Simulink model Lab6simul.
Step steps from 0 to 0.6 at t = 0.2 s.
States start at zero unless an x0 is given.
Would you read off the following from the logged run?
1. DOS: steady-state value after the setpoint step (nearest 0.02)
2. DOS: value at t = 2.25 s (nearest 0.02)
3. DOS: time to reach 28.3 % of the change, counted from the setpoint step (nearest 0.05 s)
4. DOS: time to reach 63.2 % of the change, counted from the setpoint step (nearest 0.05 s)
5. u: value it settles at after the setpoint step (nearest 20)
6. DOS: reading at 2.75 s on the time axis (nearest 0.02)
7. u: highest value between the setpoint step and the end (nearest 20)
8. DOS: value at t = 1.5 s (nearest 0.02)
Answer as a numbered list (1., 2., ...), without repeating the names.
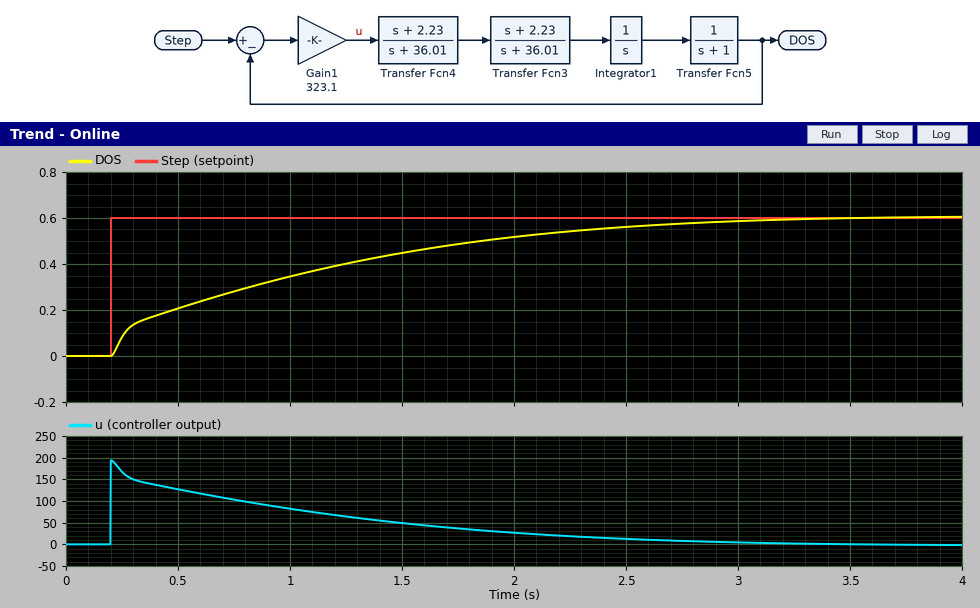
1. 0.60
2. 0.54
3. 0.20 s
4. 0.95 s
5. 0
6. 0.58
7. 200
8. 0.44
